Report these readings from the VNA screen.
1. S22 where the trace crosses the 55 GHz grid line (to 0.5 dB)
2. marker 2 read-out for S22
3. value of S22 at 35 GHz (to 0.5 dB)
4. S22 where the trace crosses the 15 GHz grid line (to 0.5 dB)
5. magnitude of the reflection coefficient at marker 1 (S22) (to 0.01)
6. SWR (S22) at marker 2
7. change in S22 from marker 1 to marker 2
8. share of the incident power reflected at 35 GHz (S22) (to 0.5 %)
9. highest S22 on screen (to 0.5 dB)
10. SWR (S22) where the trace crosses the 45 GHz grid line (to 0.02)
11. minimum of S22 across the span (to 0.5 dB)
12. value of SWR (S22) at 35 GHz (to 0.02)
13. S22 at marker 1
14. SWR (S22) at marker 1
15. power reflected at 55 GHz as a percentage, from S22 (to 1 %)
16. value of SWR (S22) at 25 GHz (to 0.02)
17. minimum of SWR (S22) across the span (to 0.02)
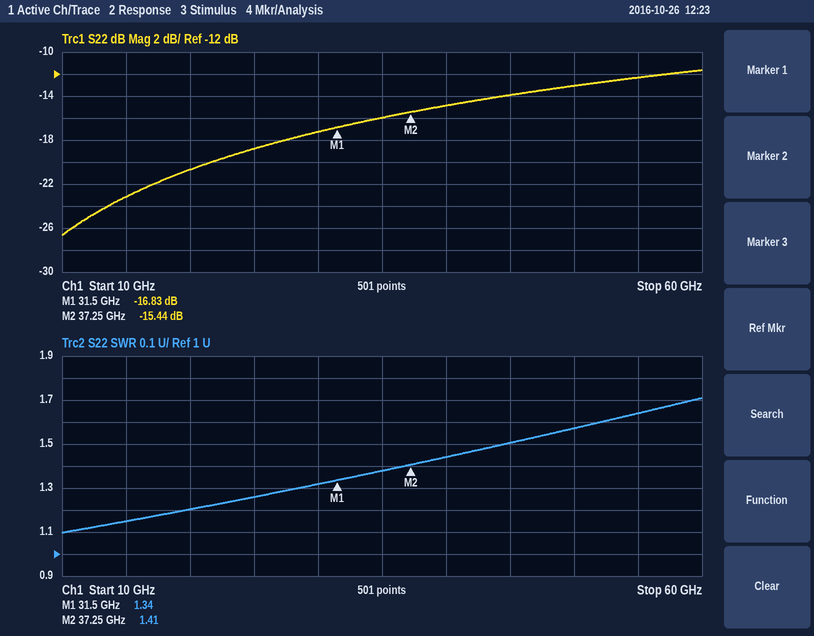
-12.5 dB
-15.44 dB
-16.0 dB
-23.0 dB
0.14
1.41
1.39 dB
2.5 %
-11.5 dB
1.50
-26.5 dB
1.38
-16.83 dB
1.34
6 %
1.26
1.10
